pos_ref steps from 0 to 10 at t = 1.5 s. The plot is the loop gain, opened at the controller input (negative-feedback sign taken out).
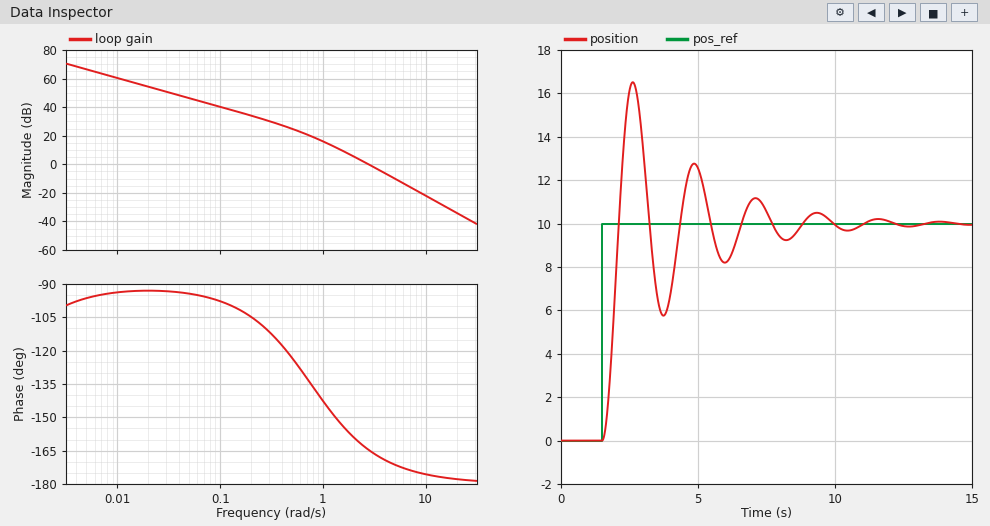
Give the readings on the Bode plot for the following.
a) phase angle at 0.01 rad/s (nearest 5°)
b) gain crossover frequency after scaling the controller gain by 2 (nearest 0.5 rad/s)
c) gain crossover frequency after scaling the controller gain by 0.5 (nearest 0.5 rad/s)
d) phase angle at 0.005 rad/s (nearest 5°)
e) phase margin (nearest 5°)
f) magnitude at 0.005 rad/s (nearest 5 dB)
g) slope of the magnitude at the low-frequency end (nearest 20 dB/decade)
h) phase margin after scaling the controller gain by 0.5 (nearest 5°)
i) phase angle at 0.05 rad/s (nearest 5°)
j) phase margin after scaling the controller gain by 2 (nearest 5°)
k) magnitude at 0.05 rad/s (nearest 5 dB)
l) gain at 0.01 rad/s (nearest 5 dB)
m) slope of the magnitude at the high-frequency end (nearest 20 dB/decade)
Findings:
-95°
4.0 rad/s
2.0 rad/s
-95°
15°
65 dB
-20 dB/decade
20°
-95°
10°
45 dB
60 dB
-40 dB/decade
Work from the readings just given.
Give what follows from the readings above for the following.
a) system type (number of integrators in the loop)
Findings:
1
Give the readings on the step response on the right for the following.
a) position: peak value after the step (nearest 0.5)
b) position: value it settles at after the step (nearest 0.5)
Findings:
16.5
10.0
